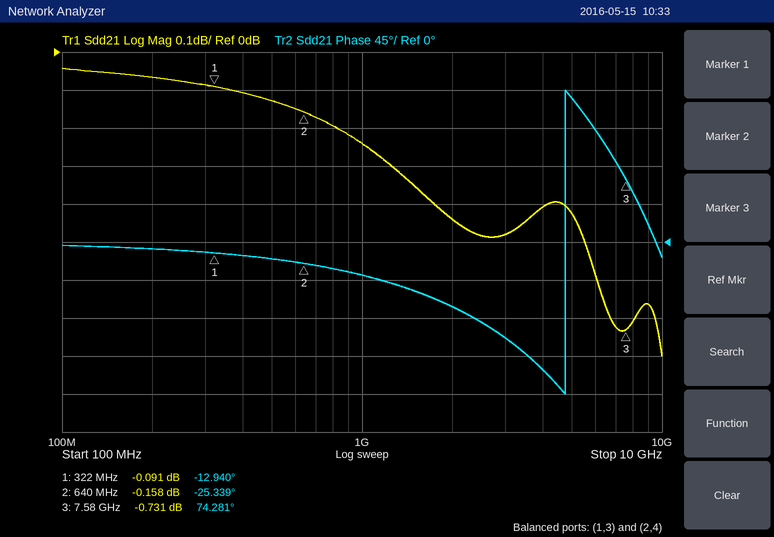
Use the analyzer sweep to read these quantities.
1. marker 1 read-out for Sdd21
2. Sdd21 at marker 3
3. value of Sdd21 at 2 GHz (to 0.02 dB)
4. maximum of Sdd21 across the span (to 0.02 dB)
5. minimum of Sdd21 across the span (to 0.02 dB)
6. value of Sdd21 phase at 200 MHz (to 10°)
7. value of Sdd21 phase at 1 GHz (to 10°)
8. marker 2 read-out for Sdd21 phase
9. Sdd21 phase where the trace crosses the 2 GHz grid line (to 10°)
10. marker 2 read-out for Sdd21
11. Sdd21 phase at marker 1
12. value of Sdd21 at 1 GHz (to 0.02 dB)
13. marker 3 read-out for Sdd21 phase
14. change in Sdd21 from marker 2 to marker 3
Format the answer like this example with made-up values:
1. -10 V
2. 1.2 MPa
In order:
1. -0.091 dB
2. -0.731 dB
3. -0.44 dB
4. -0.04 dB
5. -0.80 dB
6. -10°
7. -40°
8. -25.339°
9. -80°
10. -0.158 dB
11. -12.940°
12. -0.24 dB
13. 74.281°
14. -0.573 dB
